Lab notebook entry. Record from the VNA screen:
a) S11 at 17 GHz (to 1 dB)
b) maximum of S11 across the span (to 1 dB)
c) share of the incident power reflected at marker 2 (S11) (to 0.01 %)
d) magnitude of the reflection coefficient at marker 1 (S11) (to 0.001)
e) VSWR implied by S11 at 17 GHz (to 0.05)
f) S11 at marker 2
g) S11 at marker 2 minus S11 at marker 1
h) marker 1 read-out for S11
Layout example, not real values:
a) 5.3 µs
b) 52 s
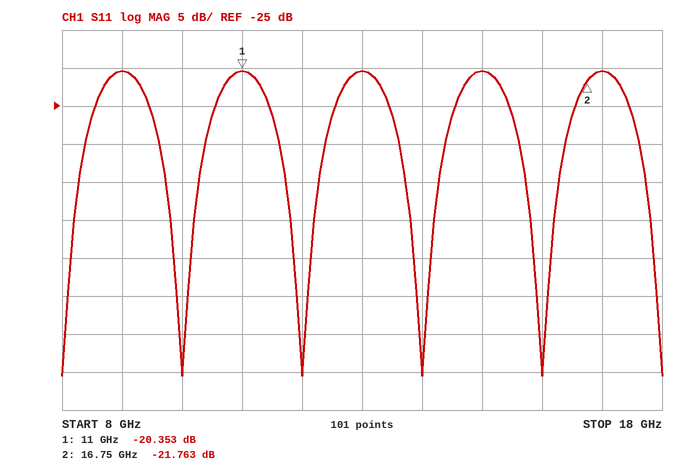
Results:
a) -20 dB
b) -20 dB
c) 0.67 %
d) 0.096
e) 1.20
f) -21.763 dB
g) -1.410 dB
h) -20.353 dB
